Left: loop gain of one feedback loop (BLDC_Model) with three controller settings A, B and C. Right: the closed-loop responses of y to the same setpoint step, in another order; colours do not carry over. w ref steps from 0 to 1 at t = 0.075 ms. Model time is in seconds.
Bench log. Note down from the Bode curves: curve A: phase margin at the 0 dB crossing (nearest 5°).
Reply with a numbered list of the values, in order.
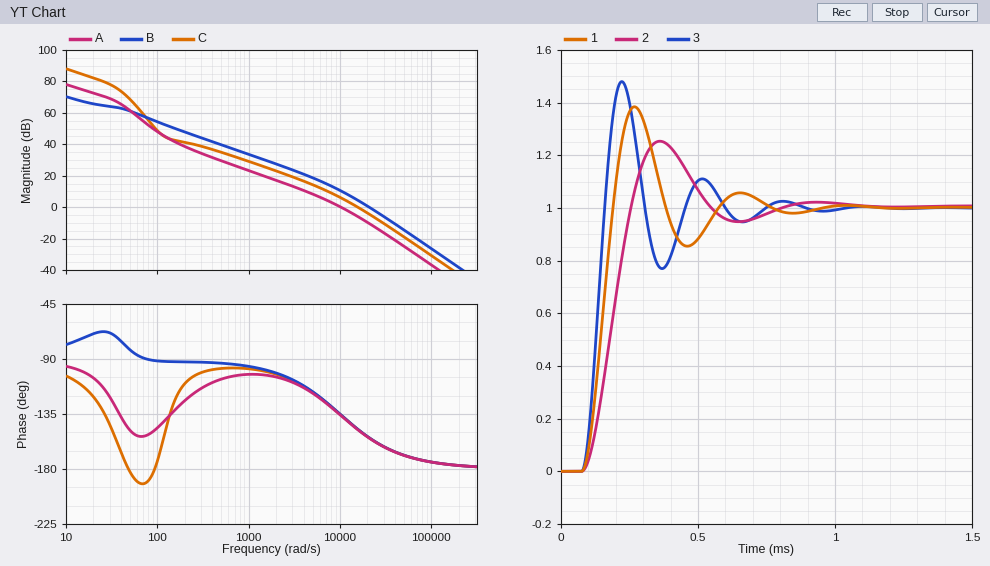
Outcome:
1. 45°
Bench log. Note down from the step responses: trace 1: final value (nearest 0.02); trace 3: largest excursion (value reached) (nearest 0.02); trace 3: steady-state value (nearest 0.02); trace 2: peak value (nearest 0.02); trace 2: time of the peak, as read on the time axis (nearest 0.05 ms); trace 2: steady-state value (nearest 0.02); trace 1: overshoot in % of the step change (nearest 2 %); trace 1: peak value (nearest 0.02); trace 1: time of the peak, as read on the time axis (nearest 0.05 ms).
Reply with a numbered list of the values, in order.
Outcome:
1. 1.00
2. 1.48
3. 1.00
4. 1.26
5. 0.35 ms
6. 1.00
7. 38 %
8. 1.38
9. 0.25 ms
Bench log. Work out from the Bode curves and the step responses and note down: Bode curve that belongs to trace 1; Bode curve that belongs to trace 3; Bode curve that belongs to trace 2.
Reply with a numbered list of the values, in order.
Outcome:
1. C
2. B
3. A
